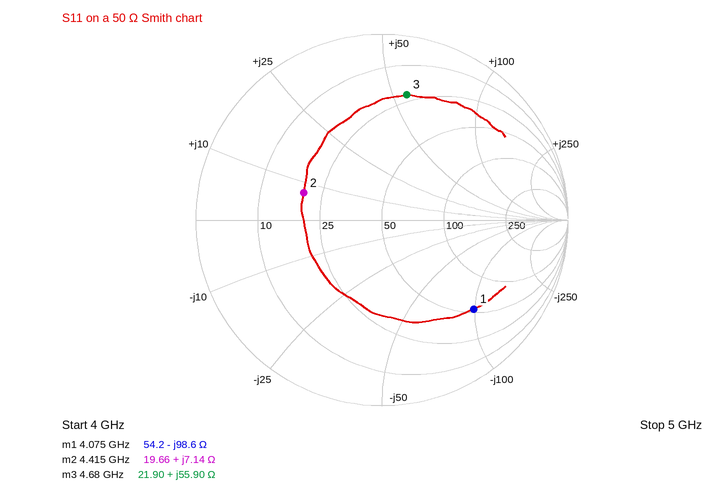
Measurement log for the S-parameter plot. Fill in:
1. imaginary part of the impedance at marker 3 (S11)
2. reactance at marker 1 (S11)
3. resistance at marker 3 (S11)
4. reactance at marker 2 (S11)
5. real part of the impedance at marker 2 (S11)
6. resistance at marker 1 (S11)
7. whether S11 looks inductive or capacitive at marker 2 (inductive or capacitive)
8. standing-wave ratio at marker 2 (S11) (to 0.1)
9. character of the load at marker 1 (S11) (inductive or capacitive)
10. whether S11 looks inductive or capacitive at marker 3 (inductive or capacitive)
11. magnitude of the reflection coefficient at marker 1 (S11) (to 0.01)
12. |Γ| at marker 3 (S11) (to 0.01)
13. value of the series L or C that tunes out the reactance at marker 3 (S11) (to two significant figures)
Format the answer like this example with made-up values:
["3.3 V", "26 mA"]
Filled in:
["+55.90 Ω", "-98.6 Ω", "21.90 Ω", "+7.14 Ω", "19.66 Ω", "54.2 Ω", "inductive", "2.6", "capacitive", "inductive", "0.69", "0.69", "610 fF"]
